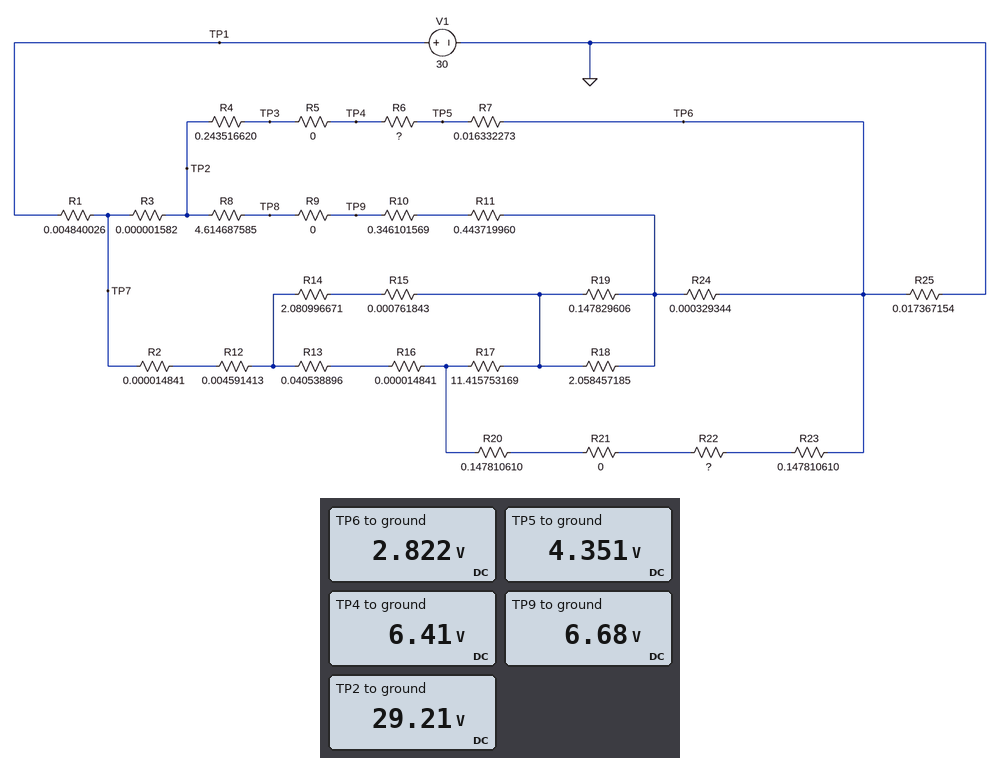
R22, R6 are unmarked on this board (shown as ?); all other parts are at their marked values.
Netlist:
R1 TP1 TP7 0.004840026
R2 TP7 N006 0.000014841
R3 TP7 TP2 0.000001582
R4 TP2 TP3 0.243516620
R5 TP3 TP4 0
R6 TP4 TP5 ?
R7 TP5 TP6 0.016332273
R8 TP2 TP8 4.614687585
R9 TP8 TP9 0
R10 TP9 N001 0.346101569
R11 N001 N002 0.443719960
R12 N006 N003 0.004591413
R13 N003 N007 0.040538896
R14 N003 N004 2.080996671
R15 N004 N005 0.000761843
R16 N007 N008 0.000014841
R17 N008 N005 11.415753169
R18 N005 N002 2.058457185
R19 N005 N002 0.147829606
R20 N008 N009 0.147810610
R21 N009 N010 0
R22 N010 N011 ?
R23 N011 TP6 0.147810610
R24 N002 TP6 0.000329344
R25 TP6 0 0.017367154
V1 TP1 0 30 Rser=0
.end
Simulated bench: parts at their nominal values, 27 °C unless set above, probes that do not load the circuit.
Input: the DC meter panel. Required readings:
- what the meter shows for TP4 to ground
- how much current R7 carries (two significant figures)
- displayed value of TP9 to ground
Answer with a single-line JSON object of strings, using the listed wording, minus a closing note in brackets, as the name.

{"what the meter shows for TP4 to ground": "6.41 V", "how much current R7 carries": "94 A", "displayed value of TP9 to ground": "6.68 V"}
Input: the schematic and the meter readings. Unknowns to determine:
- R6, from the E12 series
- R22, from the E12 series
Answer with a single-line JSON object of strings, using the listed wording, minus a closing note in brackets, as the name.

{"R6, from the E12 series": "0.022 Ω", "R22, from the E12 series": "0.18 Ω"}
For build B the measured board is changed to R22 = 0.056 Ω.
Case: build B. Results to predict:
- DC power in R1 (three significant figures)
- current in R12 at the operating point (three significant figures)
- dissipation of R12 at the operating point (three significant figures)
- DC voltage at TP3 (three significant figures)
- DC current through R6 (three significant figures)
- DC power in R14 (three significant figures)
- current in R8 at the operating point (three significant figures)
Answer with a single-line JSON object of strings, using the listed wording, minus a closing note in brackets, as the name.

{"DC power in R1": "150 W", "current in R12 at the operating point": "78.7 A", "dissipation of R12 at the operating point": "28.5 W", "DC voltage at TP3": "6.61 V", "DC current through R6": "92.6 A", "DC power in R14": "274 W", "current in R8 at the operating point": "4.83 A"}
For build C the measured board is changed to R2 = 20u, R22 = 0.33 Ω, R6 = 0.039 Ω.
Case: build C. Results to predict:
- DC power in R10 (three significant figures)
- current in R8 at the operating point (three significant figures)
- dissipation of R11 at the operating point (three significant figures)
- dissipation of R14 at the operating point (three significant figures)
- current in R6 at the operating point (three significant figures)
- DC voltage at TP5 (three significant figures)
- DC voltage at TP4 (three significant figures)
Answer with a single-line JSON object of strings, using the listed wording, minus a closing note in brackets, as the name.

{"DC power in R10": "8.46 W", "current in R8 at the operating point": "4.94 A", "dissipation of R11 at the operating point": "10.8 W", "dissipation of R14 at the operating point": "290 W", "current in R6 at the operating point": "89.4 A", "DC voltage at TP5": "4.03 V", "DC voltage at TP4": "7.51 V"}
